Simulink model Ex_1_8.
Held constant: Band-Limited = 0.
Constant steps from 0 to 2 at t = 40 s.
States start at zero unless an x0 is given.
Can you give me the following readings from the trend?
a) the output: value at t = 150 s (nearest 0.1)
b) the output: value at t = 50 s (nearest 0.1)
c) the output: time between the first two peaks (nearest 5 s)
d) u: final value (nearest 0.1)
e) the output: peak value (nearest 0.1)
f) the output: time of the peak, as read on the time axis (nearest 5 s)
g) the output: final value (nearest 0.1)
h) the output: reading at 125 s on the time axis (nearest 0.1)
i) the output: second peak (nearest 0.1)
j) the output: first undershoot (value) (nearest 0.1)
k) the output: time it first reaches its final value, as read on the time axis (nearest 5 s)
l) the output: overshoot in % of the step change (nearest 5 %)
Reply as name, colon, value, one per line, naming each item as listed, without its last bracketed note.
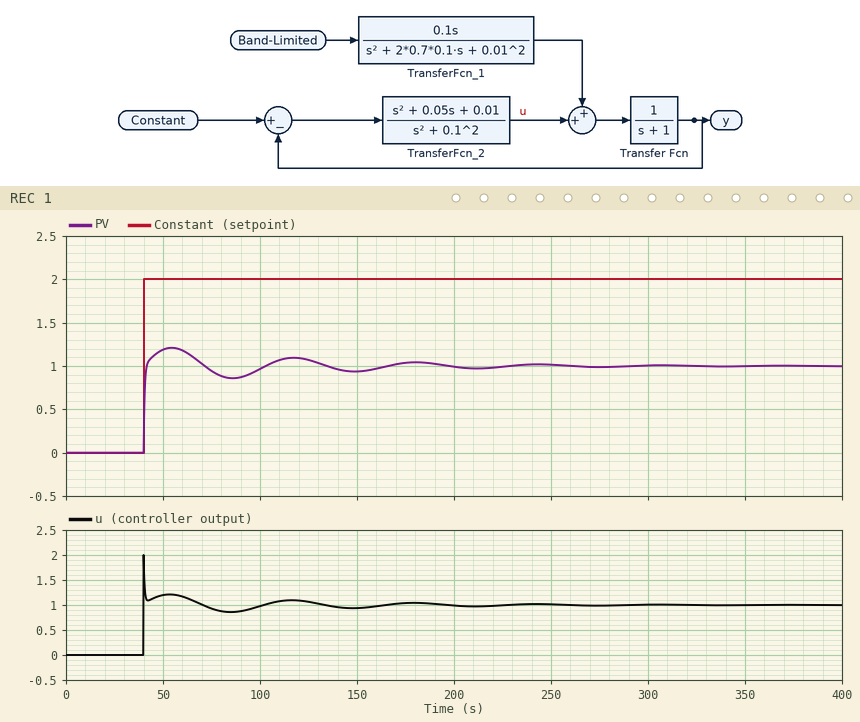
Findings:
the output: value at t = 150 s: 0.9
the output: value at t = 50 s: 1.2
the output: time between the first two peaks: 65 s
u: final value: 1.0
the output: peak value: 1.2
the output: time of the peak, as read on the time axis: 55 s
the output: final value: 1.0
the output: reading at 125 s on the time axis: 1.1
the output: second peak: 1.1
the output: first undershoot (value): 0.9
the output: time it first reaches its final value, as read on the time axis: 40 s
the output: overshoot in % of the step change: 20 %
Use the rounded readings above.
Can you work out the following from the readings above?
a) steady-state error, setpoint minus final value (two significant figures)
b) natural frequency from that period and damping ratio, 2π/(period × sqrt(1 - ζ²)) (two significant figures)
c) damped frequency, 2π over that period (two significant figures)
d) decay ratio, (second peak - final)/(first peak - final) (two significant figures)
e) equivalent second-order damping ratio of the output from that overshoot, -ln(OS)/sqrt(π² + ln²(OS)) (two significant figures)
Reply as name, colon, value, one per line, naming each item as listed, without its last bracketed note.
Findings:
steady-state error, setpoint minus final value: 1.0
natural frequency from that period and damping ratio, 2π/(period × sqrt(1 - ζ²)): 0.11 rad/s
damped frequency, 2π over that period: 0.097 rad/s
decay ratio, (second peak - final)/(first peak - final): 0.50
equivalent second-order damping ratio of the output from that overshoot, -ln(OS)/sqrt(π² + ln²(OS)): 0.46
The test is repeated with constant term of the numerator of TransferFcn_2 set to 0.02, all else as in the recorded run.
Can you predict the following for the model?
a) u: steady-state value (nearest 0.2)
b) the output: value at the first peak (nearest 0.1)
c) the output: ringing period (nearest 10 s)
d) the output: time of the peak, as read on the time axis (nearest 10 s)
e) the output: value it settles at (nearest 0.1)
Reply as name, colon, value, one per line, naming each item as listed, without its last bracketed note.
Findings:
u: steady-state value: 1.4
the output: value at the first peak: 1.6
the output: ringing period: 50 s
the output: time of the peak, as read on the time axis: 60 s
the output: value it settles at: 1.3
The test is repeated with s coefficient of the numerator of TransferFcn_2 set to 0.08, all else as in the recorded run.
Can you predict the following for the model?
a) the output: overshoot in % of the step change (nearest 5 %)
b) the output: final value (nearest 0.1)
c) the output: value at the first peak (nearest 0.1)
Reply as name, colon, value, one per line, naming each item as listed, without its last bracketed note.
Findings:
the output: overshoot in % of the step change: 30 %
the output: final value: 1.0
the output: value at the first peak: 1.3
